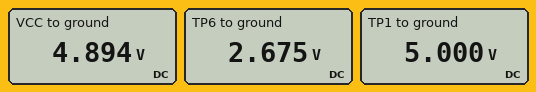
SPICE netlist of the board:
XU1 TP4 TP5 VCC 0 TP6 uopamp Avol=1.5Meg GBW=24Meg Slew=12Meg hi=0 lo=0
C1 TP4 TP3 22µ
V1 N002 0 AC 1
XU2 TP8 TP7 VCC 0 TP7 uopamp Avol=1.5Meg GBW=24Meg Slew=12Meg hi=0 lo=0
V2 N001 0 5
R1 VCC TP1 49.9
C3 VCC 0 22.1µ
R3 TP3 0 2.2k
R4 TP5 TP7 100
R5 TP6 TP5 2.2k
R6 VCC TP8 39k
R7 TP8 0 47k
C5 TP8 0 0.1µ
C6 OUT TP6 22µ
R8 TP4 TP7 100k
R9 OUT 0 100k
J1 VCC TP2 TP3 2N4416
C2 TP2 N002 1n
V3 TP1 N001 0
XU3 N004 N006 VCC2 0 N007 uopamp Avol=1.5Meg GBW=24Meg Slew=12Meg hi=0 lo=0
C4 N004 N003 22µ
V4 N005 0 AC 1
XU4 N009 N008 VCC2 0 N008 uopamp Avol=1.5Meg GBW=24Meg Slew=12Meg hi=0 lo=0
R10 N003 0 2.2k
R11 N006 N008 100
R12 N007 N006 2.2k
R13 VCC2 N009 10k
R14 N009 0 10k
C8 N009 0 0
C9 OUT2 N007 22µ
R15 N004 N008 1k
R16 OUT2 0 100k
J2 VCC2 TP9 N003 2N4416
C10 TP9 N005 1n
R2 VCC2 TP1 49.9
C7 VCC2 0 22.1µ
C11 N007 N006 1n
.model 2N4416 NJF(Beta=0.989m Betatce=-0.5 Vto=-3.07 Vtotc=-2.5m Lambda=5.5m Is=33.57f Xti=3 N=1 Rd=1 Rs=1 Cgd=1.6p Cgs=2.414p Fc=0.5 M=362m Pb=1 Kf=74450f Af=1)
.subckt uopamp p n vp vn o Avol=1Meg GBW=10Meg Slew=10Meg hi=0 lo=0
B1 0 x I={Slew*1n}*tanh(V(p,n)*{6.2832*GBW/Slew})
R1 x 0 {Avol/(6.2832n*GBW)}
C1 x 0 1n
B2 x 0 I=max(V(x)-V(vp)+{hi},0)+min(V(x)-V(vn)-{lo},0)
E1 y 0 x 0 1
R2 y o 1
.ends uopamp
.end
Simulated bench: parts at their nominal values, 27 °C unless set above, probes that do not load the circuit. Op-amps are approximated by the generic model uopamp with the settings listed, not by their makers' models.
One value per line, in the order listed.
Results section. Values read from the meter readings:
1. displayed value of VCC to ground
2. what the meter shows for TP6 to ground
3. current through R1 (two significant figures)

4.894 V
2.675 V
2.1 mA
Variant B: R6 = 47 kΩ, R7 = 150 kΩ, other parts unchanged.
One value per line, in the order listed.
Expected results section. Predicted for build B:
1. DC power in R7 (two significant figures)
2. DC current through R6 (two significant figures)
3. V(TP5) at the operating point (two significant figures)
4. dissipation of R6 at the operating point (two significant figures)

93 µW
25 µA
3.7 V
29 µW
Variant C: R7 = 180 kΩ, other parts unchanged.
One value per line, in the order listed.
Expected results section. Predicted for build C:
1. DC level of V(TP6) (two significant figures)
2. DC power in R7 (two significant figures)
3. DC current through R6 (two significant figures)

4.0 V
90 µW
22 µA
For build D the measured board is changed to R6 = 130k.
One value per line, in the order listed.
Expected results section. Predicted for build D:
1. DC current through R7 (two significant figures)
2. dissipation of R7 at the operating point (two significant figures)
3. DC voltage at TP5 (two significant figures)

28 µA
36 µW
1.3 V
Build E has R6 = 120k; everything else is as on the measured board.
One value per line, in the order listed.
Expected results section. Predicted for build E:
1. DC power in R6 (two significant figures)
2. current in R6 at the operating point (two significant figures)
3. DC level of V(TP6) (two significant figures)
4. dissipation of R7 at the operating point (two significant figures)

100 µW
29 µA
1.4 V
40 µW
